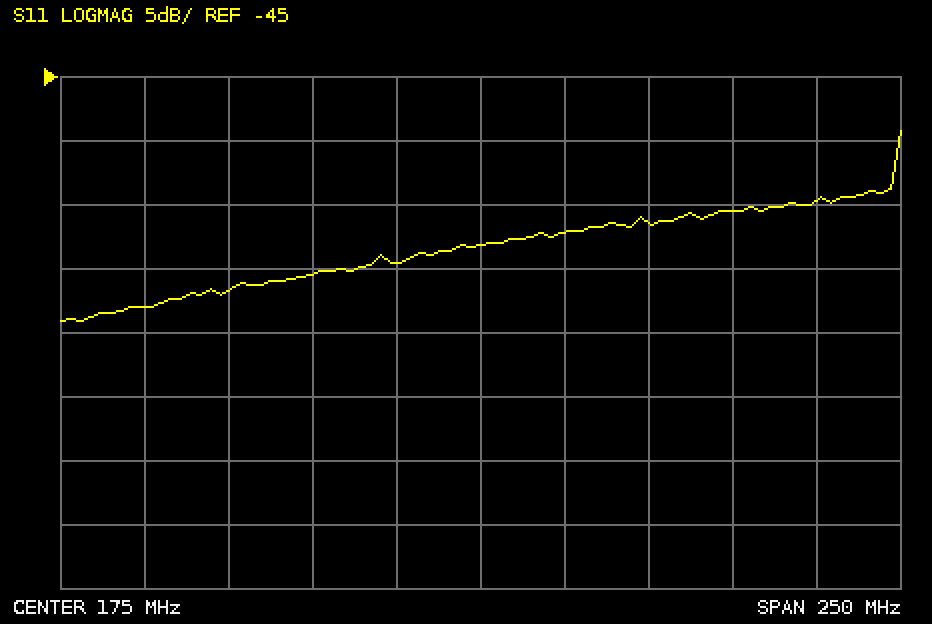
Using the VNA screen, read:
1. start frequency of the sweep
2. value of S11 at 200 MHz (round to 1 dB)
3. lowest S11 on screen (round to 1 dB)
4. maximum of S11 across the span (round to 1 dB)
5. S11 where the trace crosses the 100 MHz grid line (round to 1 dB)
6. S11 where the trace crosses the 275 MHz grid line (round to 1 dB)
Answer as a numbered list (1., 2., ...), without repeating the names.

1. 50 MHz
2. -57 dB
3. -64 dB
4. -49 dB
5. -62 dB
6. -55 dB
